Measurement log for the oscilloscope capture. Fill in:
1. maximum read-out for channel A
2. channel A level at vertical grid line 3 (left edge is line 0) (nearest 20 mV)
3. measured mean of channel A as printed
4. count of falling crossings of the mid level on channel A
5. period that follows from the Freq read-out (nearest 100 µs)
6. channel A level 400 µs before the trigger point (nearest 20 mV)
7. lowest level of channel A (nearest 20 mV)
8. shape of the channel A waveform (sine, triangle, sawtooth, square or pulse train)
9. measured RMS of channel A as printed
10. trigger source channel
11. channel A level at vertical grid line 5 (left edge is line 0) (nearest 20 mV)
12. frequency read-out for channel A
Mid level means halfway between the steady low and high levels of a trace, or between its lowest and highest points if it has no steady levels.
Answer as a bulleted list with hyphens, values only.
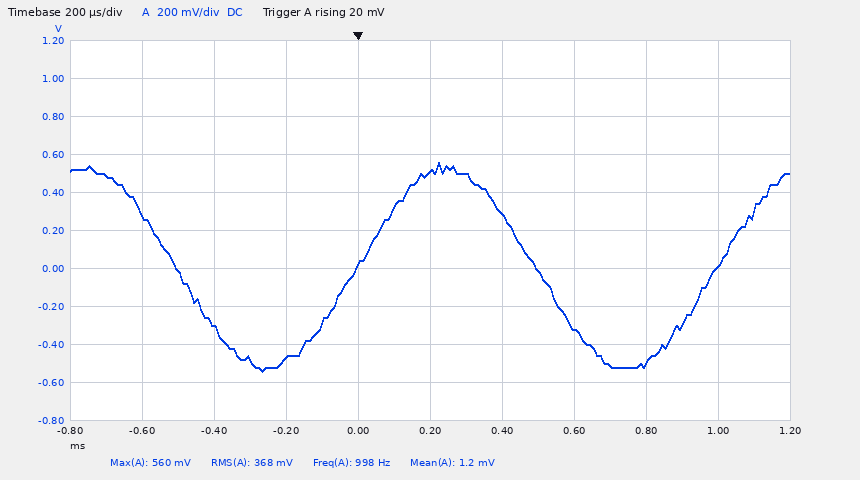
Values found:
- 560 mV
- -480 mV
- 1.2 mV
- 2
- 1.0 ms
- -300 mV
- -540 mV
- sine
- 368 mV
- channel A
- 500 mV
- 998 Hz
